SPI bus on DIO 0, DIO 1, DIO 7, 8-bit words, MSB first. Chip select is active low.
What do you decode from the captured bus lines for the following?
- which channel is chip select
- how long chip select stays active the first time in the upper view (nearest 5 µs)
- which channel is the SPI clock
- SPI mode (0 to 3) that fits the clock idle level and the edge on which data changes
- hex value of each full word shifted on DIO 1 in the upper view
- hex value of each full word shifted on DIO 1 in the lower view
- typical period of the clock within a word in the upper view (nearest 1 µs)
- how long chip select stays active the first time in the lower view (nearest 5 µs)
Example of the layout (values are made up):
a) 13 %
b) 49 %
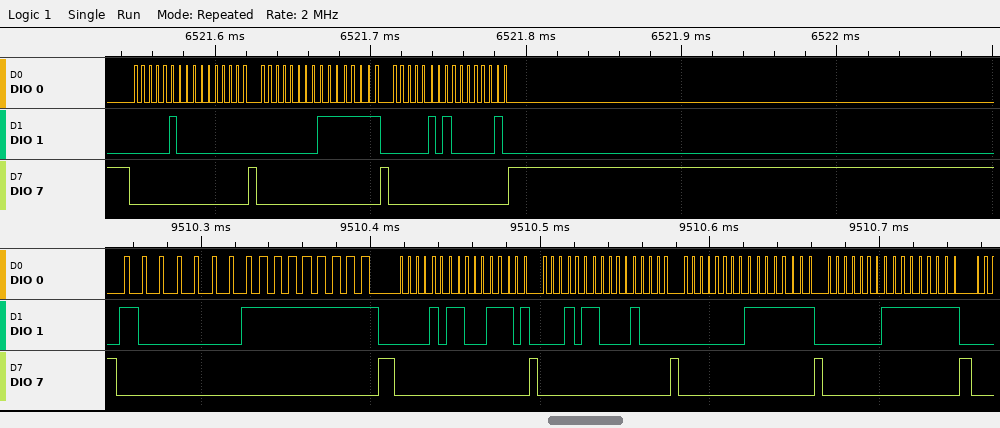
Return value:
a) DIO 7
b) 75 µs
c) DIO 0
d) 1
e) 04, 00, 00, FF, 05, 02
f) 81, FF, 0B, 1D, 16, 10, 00, FF, 01, FF
g) 5 µs
h) 155 µs
